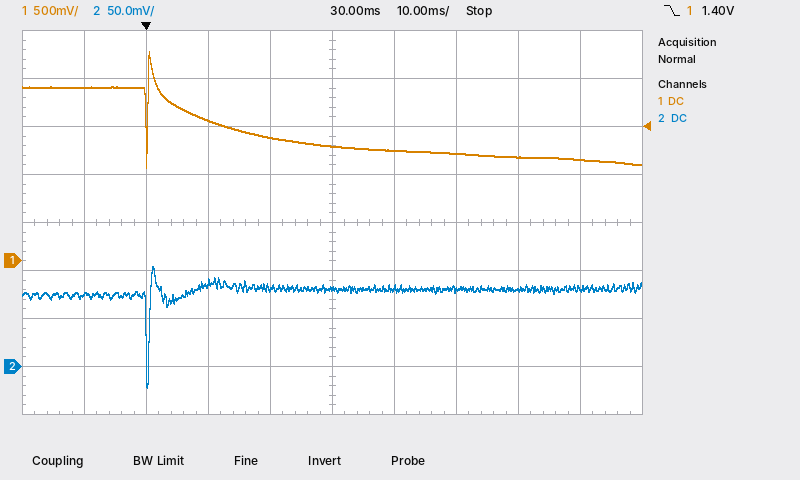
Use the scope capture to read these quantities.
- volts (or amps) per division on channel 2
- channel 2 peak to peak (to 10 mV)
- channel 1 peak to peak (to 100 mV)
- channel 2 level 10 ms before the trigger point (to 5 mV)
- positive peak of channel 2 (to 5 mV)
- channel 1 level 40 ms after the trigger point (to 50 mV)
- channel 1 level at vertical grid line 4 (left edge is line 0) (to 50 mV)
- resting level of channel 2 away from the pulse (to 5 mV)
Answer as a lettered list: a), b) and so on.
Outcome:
a) 50 mV
b) 130 mV
c) 1.20 V
d) 75 mV
e) 105 mV
f) 1.15 V
g) 1.30 V
h) 80 mV
